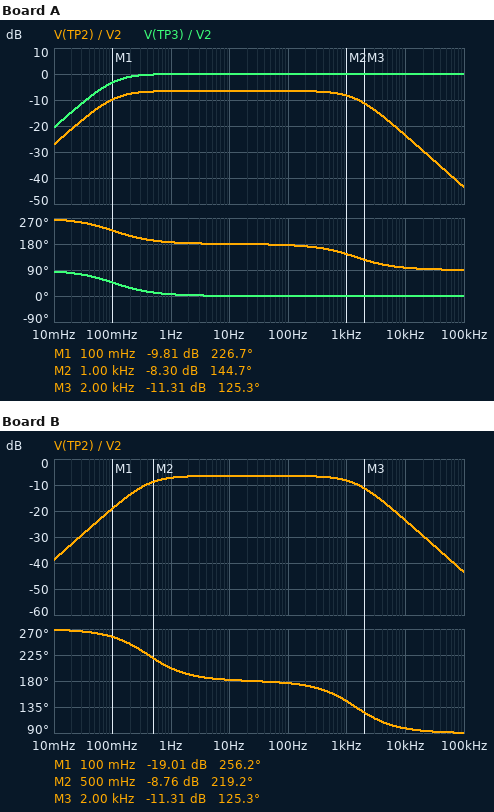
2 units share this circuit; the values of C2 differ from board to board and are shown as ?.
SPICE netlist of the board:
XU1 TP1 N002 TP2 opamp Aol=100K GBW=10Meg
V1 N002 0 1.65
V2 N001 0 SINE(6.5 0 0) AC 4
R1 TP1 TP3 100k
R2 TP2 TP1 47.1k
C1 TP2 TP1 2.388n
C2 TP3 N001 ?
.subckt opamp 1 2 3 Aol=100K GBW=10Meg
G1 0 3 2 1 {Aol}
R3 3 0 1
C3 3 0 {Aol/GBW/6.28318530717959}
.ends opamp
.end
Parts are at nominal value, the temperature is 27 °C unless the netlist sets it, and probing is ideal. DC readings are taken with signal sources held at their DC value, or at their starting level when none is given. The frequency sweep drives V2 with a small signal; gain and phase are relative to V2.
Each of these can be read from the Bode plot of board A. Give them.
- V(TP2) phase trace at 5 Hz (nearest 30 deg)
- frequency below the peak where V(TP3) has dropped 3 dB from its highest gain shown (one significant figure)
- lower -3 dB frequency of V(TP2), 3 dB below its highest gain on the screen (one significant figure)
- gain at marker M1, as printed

180 deg
100 mHz
100 mHz
-9.81 dB
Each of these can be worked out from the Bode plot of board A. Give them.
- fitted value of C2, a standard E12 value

15 µF
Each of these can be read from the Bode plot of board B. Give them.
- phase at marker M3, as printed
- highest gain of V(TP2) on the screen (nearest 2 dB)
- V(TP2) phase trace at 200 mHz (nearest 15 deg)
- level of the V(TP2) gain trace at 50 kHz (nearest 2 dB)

125.3 deg
-6 dB
240 deg
-38 dB
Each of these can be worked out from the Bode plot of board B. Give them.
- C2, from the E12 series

3.9 µF
